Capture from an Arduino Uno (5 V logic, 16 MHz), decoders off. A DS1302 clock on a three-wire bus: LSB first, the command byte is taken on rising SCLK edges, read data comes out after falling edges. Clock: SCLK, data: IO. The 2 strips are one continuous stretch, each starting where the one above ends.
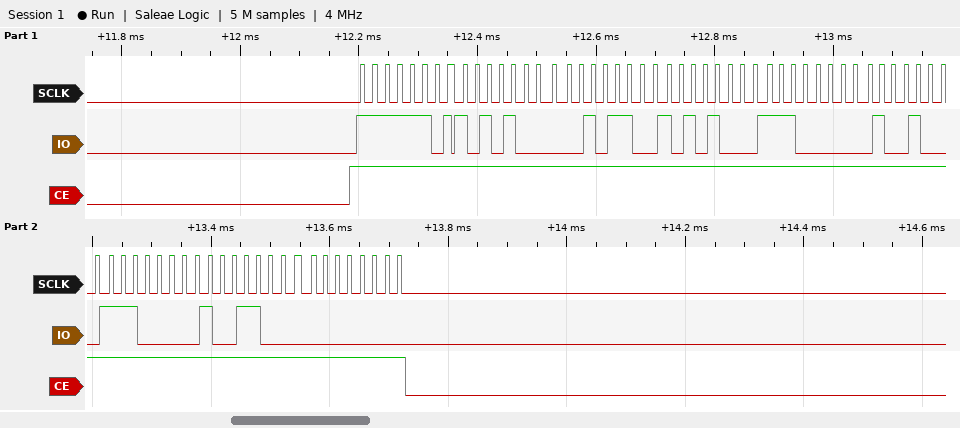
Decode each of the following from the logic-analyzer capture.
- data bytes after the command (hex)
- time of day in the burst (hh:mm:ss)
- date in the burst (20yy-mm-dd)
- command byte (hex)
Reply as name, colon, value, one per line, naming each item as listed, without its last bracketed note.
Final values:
data bytes after the command: 15 34 15 07 12 07 19 00
time of day in the burst: 15:34:15
date in the burst: 2019-12-07
command byte: 0xBF
